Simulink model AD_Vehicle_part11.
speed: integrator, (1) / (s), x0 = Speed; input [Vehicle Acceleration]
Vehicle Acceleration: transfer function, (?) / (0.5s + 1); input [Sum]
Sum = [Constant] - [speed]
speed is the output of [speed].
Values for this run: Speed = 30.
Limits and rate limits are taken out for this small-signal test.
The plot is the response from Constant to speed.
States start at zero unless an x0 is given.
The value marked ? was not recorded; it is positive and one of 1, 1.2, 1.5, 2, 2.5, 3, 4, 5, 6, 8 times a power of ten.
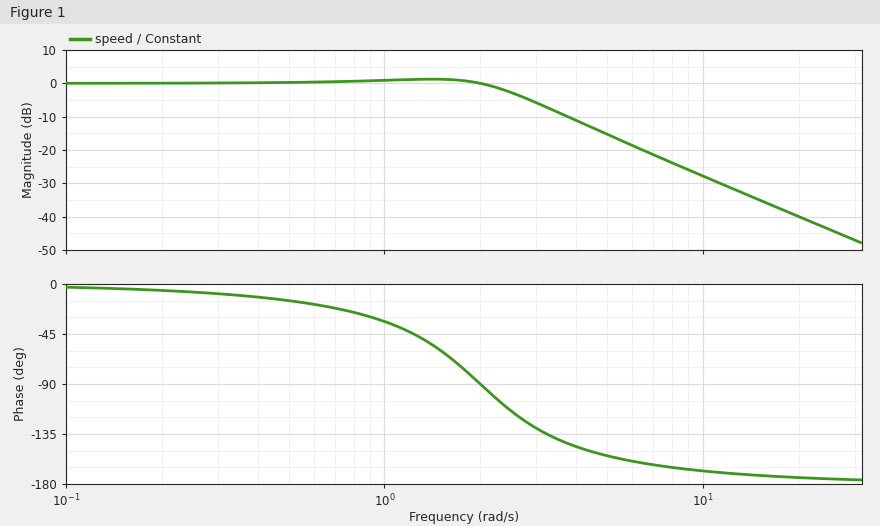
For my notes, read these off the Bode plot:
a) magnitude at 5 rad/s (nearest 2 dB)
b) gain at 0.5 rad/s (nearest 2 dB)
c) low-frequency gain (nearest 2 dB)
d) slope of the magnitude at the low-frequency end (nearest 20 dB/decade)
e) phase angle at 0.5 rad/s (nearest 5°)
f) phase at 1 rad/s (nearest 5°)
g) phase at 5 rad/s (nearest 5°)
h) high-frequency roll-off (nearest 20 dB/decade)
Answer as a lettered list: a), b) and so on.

a) -16 dB
b) 0 dB
c) 0 dB
d) 0 dB/decade
e) -15°
f) -35°
g) -155°
h) -40 dB/decade
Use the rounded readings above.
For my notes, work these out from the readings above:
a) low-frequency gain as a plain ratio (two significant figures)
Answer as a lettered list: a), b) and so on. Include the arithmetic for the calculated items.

a) 10^(0 / 20) = 1.0
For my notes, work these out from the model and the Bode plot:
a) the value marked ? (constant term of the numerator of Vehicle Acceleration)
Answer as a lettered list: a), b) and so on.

a) 2
